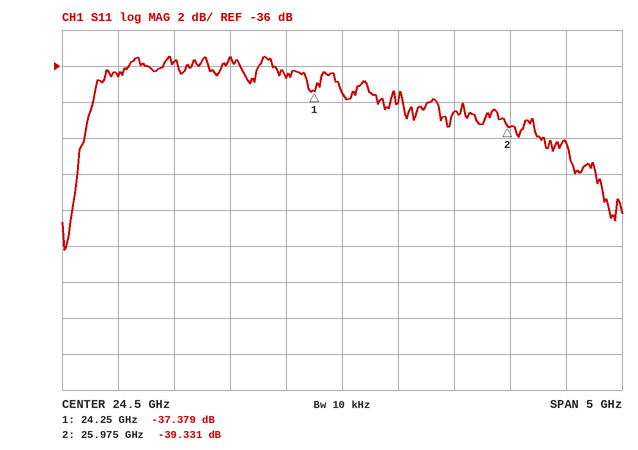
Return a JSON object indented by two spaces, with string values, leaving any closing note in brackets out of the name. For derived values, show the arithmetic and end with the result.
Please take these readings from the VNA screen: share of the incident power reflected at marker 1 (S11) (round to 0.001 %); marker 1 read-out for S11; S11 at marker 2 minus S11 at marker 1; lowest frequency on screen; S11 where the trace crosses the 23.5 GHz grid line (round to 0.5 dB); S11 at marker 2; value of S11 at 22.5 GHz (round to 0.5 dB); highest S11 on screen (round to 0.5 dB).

{
  "share of the incident power reflected at marker 1 (S11)": "10^(-37.379/10) ≈ 0.018 %",
  "marker 1 read-out for S11": "-37.379 dB",
  "S11 at marker 2 minus S11 at marker 1": "-39.331 − (-37.379) = -1.952 dB",
  "lowest frequency on screen": "22 GHz",
  "S11 where the trace crosses the 23.5 GHz grid line": "-35.5 dB",
  "S11 at marker 2": "-39.331 dB",
  "value of S11 at 22.5 GHz": "-36.5 dB",
  "highest S11 on screen": "-35.5 dB"
}
